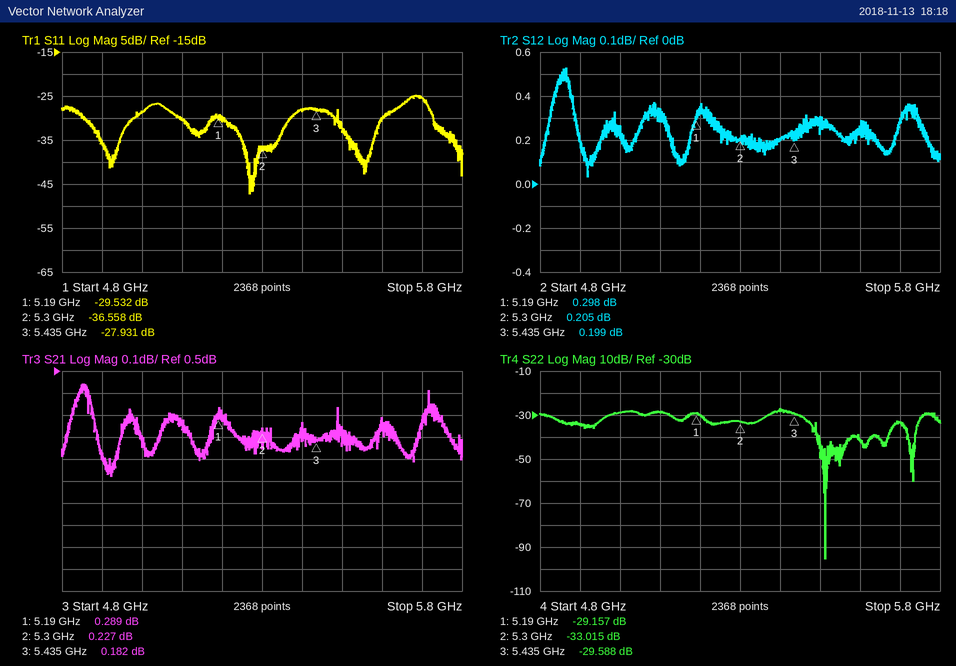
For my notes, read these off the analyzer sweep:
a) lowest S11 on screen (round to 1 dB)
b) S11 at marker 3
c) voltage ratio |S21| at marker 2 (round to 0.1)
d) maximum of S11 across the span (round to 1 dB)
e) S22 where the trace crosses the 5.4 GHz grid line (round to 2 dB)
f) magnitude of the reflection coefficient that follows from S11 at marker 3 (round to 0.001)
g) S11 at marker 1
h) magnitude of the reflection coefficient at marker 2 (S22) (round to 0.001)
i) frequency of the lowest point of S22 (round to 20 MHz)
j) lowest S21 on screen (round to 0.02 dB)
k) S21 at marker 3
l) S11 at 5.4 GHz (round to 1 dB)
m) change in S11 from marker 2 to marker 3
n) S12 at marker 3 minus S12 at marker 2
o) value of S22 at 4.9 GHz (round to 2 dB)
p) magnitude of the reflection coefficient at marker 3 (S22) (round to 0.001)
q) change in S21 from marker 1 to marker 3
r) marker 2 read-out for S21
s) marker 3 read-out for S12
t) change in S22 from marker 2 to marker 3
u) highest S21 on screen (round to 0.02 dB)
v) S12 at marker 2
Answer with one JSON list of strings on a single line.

["-47 dB", "-27.931 dB", "1.0", "-25 dB", "-28 dB", "0.040", "-29.532 dB", "0.022", "5.52 GHz", "0.02 dB", "0.182 dB", "-28 dB", "8.627 dB", "-0.006 dB", "-34 dB", "0.033", "-0.107 dB", "0.227 dB", "0.199 dB", "3.427 dB", "0.44 dB", "0.205 dB"]
